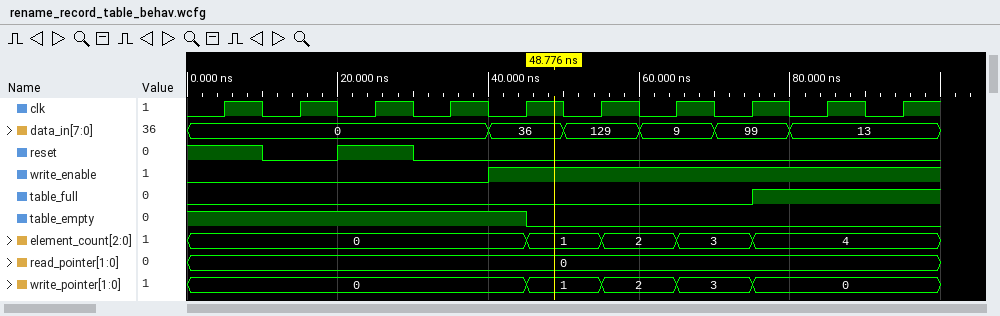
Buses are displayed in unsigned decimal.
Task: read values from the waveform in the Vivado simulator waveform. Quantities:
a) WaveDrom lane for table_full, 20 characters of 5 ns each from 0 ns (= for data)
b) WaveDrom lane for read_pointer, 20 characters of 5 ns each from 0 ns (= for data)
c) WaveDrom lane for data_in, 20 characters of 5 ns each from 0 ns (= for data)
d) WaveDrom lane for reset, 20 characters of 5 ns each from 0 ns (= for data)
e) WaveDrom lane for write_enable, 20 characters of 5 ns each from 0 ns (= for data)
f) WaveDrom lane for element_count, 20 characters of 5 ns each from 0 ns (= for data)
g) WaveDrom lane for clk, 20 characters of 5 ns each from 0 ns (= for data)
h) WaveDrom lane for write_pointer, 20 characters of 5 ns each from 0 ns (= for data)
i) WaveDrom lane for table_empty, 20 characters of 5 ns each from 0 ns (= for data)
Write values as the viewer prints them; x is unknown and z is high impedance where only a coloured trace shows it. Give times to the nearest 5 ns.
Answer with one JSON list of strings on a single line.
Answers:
["{name: 'table_full', wave: '0..............1....'}", "{name: 'read_pointer', wave: '=...................', data: '0'}", "{name: 'data_in', wave: '=.......=.=.=.=.=...', data: '0 36 129 9 99 13'}", "{name: 'reset', wave: '1.0.1.0.............'}", "{name: 'write_enable', wave: '0.......1...........'}", "{name: 'element_count', wave: '=........=.=.=.=....', data: '0 1 2 3 4'}", "{name: 'clk', wave: '01010101010101010101'}", "{name: 'write_pointer', wave: '=........=.=.=.=....', data: '0 1 2 3 0'}", "{name: 'table_empty', wave: '1........0..........'}"]
